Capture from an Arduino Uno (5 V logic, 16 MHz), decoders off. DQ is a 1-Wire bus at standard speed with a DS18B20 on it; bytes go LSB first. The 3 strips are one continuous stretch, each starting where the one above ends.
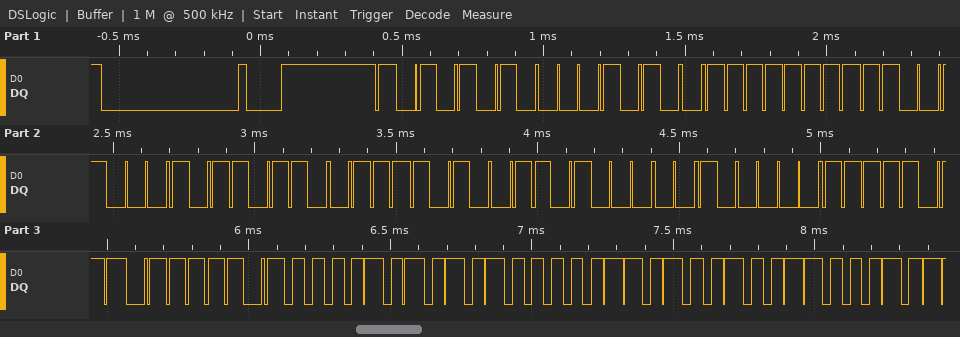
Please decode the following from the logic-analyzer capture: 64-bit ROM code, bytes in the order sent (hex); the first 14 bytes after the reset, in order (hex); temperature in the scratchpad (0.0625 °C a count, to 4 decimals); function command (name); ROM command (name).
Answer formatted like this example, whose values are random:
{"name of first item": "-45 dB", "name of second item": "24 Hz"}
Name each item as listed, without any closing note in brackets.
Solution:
{"64-bit ROM code, bytes in the order sent": "28 FF 13 6D 5E 16 04 DF", "the first 14 bytes after the reset, in order": "55 28 FF 13 6D 5E 16 04 DF BE 50 05 4B 46", "temperature in the scratchpad": "85.0000 °C", "function command": "Read Scratchpad", "ROM command": "Match ROM"}
